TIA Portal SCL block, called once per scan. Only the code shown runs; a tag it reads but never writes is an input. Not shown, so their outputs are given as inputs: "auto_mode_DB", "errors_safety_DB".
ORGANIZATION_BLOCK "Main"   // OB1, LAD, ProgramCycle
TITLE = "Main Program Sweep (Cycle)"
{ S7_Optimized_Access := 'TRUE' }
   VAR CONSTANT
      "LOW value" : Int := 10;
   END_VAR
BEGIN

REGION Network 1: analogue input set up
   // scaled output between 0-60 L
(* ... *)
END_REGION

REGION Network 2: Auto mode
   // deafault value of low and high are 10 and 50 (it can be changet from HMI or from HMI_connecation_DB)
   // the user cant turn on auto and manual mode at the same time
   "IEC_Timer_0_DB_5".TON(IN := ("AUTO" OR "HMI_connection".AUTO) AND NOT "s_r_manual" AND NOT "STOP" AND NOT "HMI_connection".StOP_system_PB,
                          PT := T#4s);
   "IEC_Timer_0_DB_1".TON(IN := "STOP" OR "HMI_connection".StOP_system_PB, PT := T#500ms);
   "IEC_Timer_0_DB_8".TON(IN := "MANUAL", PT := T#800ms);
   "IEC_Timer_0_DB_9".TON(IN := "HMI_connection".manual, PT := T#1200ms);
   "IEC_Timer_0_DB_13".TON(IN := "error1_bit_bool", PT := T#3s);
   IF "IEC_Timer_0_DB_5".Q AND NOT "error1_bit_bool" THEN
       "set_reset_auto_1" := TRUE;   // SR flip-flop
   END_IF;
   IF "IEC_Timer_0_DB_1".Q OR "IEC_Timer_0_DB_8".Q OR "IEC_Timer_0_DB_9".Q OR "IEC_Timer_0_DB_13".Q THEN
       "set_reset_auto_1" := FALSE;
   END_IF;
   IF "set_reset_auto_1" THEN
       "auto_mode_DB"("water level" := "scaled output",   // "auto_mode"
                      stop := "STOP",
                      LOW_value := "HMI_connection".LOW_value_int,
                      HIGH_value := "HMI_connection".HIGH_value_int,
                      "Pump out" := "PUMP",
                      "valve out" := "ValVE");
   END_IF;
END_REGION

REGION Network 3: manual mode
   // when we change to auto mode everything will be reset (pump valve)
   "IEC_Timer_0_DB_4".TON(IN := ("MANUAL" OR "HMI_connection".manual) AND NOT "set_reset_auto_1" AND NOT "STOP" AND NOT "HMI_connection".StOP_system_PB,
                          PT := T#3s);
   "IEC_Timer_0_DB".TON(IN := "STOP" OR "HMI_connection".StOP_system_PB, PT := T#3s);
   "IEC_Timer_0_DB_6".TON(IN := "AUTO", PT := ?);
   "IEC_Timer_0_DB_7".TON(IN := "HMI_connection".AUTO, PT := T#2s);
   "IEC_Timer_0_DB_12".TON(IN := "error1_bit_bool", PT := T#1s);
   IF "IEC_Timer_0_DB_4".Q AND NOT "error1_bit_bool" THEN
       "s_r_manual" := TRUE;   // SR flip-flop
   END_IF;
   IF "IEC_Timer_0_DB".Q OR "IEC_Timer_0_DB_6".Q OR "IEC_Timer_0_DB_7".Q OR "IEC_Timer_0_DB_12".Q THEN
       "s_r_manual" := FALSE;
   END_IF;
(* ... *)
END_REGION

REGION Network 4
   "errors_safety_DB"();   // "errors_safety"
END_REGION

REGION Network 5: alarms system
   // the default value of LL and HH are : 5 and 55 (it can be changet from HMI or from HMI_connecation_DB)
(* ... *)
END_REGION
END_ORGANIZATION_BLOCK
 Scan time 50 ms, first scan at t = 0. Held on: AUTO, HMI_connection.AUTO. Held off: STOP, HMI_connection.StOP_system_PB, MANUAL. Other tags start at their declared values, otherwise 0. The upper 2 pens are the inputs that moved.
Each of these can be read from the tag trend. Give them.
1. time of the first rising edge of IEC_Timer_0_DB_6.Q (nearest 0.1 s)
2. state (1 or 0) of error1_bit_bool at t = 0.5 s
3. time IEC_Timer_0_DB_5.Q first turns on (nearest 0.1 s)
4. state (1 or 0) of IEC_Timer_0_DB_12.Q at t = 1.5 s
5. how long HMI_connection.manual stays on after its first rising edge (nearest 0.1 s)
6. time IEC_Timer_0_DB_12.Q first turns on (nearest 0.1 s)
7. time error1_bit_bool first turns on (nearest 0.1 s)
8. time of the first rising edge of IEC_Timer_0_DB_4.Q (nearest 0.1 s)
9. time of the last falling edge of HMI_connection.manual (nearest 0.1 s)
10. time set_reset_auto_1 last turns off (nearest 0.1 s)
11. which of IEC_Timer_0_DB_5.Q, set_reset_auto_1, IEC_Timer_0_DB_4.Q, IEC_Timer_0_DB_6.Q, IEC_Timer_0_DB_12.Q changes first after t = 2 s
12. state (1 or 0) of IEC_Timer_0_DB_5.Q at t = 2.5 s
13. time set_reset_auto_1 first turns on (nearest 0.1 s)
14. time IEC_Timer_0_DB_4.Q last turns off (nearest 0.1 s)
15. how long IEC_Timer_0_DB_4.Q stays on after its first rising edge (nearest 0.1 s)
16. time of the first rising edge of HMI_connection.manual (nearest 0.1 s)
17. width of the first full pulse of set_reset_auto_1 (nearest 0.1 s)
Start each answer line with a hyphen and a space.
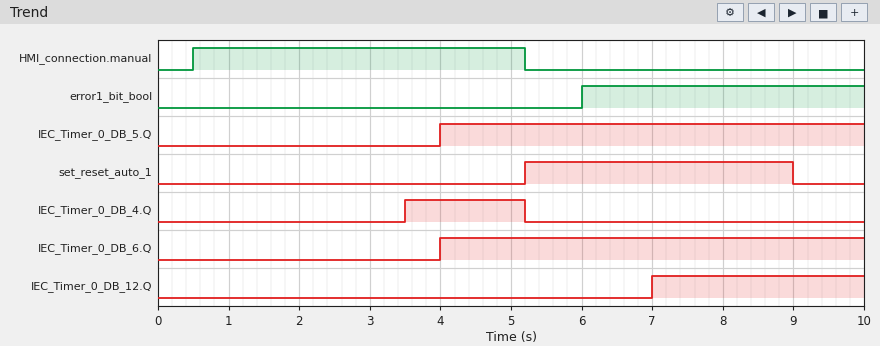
- 4.0 s
- 0
- 4.0 s
- 0
- 4.7 s
- 7.0 s
- 6.0 s
- 3.5 s
- 5.2 s
- 9.0 s
- IEC_Timer_0_DB_4.Q
- 0
- 5.2 s
- 5.2 s
- 1.7 s
- 0.5 s
- 3.8 s
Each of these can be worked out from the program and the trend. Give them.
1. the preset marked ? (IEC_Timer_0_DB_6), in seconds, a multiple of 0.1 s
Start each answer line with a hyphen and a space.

- 4.0 s
